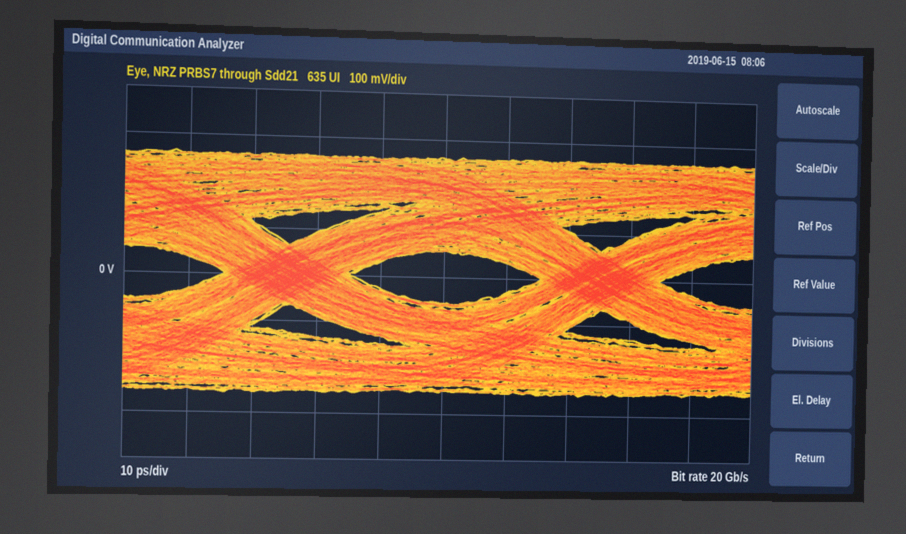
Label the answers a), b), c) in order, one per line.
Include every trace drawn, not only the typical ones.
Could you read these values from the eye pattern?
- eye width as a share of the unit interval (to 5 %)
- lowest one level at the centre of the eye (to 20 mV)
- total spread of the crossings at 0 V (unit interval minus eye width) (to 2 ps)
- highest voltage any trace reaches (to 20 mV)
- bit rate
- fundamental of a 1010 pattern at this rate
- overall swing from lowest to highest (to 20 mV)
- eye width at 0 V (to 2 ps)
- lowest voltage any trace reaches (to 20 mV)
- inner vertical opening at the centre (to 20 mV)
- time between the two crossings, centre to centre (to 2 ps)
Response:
a) 60 %
b) 60 mV
c) 20 ps
d) 260 mV
e) 20 Gb/s
f) 10 GHz
g) 520 mV
h) 30 ps
i) -260 mV
j) 120 mV
k) 50 ps
